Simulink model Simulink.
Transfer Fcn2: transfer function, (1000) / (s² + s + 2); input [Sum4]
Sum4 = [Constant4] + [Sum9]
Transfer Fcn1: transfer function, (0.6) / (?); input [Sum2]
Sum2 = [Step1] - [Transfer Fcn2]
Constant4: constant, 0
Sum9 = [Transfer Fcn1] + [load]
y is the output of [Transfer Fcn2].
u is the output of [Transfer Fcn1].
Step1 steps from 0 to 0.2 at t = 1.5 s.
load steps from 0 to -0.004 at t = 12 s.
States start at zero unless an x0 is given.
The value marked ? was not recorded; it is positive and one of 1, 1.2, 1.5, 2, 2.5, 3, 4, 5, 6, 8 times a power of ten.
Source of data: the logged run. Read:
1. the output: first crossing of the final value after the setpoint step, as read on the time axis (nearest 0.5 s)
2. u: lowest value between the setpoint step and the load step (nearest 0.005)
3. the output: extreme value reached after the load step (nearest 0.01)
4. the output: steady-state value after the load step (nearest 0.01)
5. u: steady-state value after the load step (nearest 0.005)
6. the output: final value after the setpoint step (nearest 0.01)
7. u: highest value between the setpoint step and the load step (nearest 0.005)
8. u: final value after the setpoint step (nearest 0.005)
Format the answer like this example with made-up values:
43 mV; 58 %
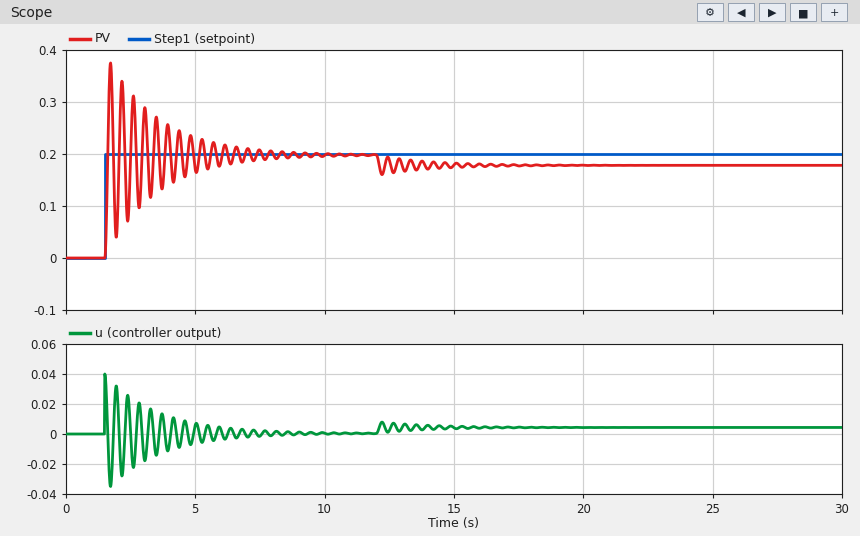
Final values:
1.5 s; -0.035; 0.16; 0.18; 0.005; 0.20; 0.040; 0.000
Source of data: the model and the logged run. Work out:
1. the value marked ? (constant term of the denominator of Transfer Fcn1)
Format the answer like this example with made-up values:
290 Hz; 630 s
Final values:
3
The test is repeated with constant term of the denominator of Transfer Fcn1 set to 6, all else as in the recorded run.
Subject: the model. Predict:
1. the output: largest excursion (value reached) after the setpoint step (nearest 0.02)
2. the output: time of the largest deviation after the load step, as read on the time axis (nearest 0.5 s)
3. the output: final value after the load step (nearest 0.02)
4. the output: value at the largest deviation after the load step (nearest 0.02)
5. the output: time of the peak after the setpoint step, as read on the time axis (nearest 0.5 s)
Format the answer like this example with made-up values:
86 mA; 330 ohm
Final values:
0.36; 12.5 s; 0.16; 0.12; 2.0 s
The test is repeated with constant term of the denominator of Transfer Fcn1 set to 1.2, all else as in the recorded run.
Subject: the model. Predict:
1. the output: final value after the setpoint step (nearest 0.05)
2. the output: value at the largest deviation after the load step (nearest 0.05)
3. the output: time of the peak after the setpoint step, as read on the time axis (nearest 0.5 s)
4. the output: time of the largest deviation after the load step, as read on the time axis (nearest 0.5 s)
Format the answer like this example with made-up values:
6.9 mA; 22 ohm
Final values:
0.20; 0.20; 1.5 s; 12.0 s
